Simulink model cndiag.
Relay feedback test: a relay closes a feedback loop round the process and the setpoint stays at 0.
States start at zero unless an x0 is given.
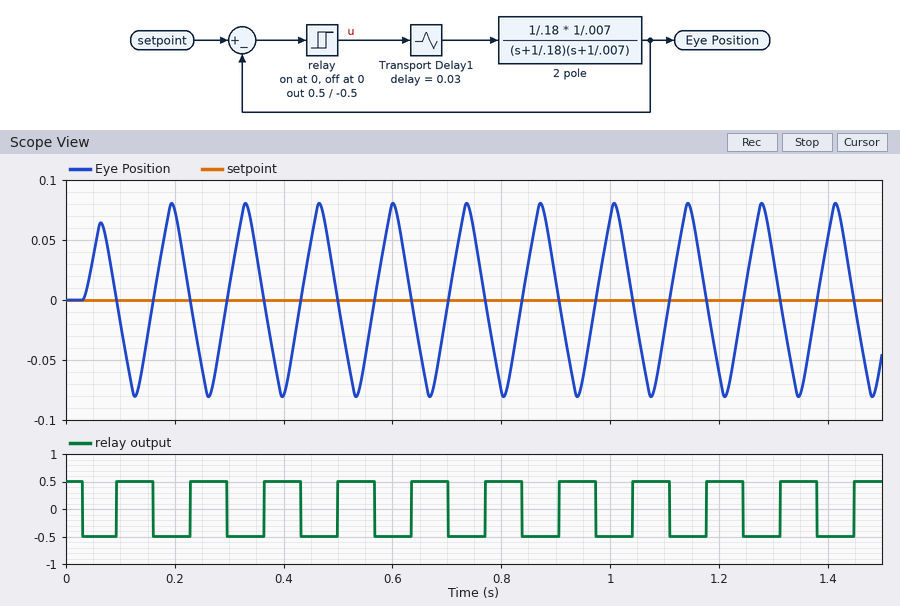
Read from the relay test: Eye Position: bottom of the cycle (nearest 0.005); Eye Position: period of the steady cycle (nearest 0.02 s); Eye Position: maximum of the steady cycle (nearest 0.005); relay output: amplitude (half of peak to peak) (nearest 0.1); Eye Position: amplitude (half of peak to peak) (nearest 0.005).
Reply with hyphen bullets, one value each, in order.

- -0.080
- 0.14 s
- 0.080
- 0.5
- 0.080
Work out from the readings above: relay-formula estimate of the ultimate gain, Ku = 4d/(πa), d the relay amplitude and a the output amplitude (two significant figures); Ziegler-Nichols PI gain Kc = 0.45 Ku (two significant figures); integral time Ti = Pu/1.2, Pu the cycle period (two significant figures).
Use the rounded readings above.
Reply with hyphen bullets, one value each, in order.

- 8.0
- 3.6
- 0.12 s
